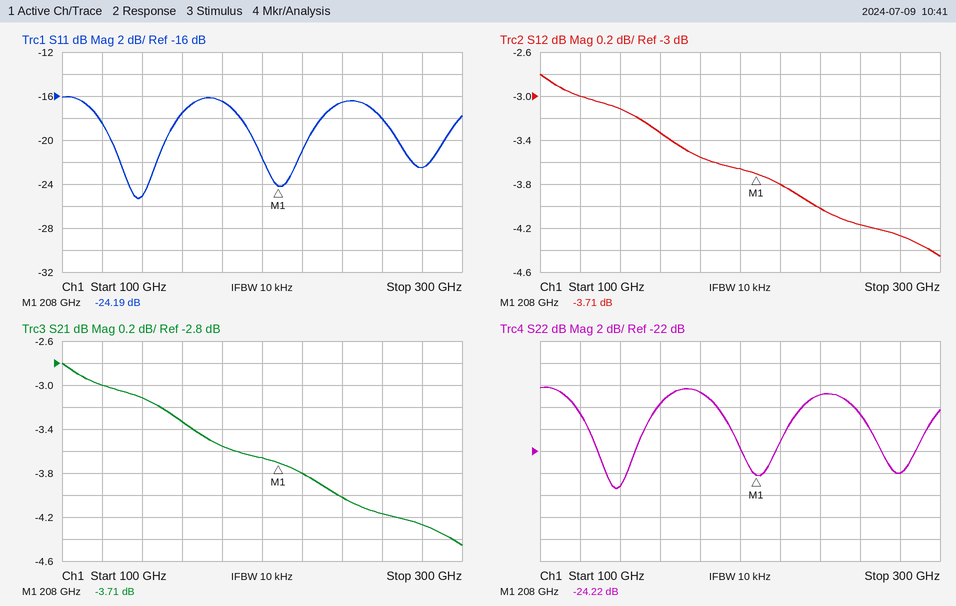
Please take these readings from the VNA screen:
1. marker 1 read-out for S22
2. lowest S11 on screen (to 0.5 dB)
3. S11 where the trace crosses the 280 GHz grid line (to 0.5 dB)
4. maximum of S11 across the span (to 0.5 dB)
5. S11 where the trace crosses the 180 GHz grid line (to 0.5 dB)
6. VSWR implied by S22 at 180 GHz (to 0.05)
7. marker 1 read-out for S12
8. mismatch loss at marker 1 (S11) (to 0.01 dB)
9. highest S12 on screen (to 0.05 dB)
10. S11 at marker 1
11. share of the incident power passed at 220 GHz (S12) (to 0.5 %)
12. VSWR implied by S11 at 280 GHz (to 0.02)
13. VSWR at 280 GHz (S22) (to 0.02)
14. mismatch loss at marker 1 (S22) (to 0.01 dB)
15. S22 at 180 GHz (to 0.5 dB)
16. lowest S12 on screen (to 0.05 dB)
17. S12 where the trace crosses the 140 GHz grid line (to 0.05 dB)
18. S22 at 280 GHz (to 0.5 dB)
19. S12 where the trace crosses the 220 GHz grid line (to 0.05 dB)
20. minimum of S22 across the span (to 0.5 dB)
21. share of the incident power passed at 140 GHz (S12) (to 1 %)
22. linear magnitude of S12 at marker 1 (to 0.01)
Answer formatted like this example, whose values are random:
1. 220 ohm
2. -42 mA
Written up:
1. -24.22 dB
2. -25.5 dB
3. -22.5 dB
4. -16.0 dB
5. -16.5 dB
6. 1.35
7. -3.71 dB
8. 0.02 dB
9. -2.80 dB
10. -24.19 dB
11. 41.5 %
12. 1.16
13. 1.14
14. 0.02 dB
15. -16.5 dB
16. -4.45 dB
17. -3.10 dB
18. -24.0 dB
19. -3.80 dB
20. -25.5 dB
21. 49 %
22. 0.65
